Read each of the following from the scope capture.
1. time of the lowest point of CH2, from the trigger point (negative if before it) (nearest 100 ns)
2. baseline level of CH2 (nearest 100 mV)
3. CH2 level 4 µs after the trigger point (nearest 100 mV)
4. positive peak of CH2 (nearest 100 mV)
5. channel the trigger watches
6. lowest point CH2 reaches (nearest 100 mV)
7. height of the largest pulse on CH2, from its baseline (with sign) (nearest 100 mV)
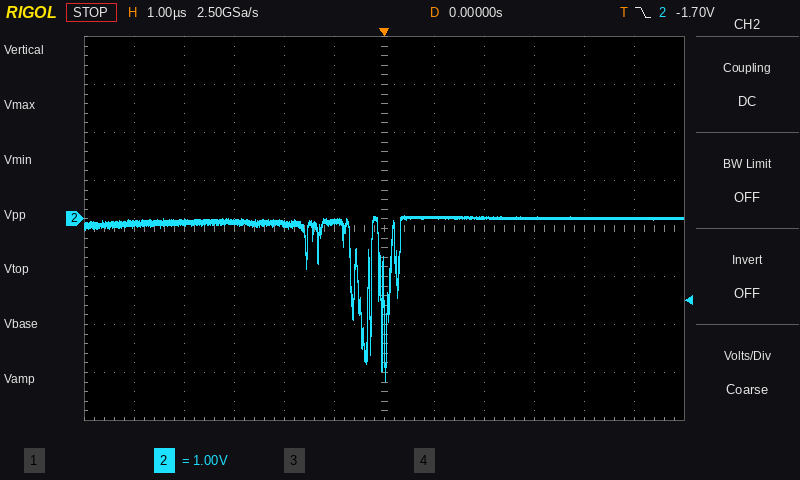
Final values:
0.0 µs
0.0 V
0.0 V
100 mV
CH2
-3.4 V
-3.4 V
